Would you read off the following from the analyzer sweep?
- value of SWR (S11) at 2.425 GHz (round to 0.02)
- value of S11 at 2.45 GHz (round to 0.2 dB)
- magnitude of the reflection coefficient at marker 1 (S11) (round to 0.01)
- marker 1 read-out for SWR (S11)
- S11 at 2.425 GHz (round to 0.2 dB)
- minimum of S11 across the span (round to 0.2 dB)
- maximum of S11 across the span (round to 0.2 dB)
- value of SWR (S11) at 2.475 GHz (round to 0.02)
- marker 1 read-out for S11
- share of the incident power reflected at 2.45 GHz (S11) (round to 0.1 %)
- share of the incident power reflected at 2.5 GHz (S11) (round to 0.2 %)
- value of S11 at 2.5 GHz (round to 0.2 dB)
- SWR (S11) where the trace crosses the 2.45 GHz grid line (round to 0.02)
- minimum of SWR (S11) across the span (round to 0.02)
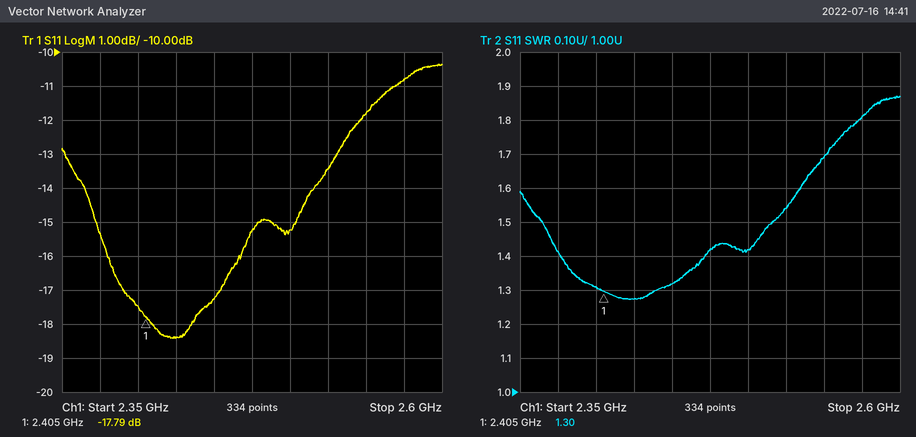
1.28
-17.2 dB
0.13
1.30
-18.4 dB
-18.4 dB
-10.4 dB
1.42
-17.79 dB
1.9 %
3.0 %
-15.2 dB
1.32
1.28
